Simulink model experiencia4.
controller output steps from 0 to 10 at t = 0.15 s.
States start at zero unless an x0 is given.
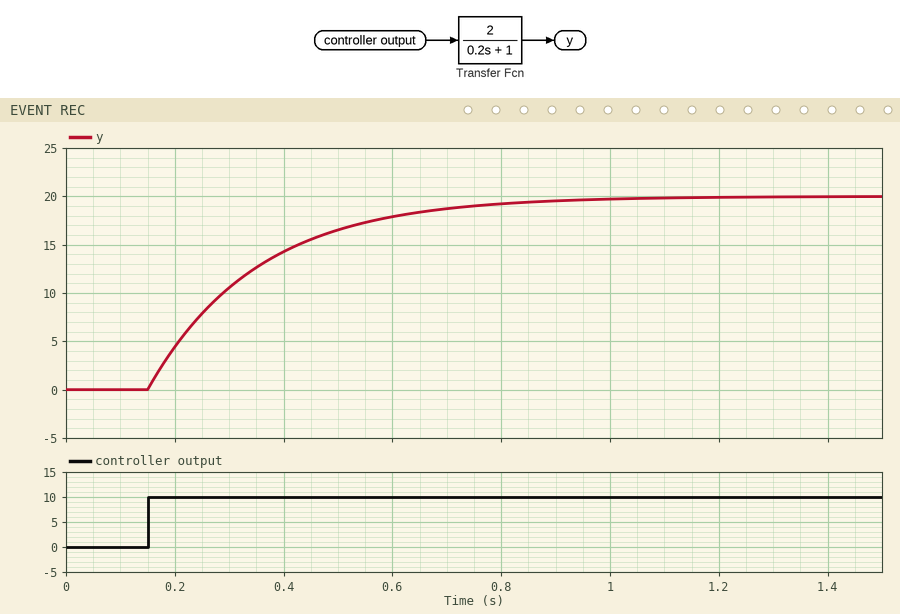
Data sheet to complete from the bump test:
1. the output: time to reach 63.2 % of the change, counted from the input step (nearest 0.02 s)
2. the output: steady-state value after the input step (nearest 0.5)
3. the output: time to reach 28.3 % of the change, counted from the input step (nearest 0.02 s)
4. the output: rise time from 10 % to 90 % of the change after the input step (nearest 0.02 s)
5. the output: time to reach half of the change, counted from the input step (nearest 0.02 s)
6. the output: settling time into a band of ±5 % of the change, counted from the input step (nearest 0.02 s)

0.20 s
20.0
0.06 s
0.44 s
0.14 s
0.60 s
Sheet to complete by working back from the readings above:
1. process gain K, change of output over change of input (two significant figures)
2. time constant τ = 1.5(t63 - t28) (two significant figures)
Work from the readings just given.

2.0
0.21 s
